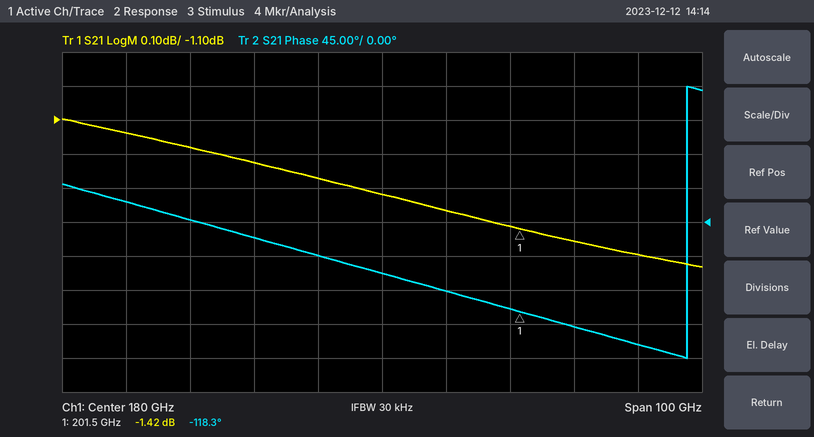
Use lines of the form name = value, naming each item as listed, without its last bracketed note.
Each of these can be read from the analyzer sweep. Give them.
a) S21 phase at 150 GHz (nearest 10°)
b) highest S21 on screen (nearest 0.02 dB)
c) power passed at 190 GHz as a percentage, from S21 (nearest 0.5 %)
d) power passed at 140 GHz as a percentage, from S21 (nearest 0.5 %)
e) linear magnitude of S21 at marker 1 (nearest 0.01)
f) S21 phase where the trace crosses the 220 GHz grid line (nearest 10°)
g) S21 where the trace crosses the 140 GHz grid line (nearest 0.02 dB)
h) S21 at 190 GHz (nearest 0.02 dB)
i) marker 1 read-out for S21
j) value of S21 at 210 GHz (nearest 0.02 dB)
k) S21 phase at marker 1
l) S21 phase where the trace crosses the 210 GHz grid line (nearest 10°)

S21 phase at 150 GHz = 0°
highest S21 on screen = -1.10 dB
power passed at 190 GHz as a percentage, from S21 = 73.0 %
power passed at 140 GHz as a percentage, from S21 = 77.0 %
linear magnitude of S21 at marker 1 = 0.85
S21 phase where the trace crosses the 220 GHz grid line = -160°
S21 where the trace crosses the 140 GHz grid line = -1.14 dB
S21 at 190 GHz = -1.36 dB
marker 1 read-out for S21 = -1.42 dB
value of S21 at 210 GHz = -1.46 dB
S21 phase at marker 1 = -118.3°
S21 phase where the trace crosses the 210 GHz grid line = -140°
